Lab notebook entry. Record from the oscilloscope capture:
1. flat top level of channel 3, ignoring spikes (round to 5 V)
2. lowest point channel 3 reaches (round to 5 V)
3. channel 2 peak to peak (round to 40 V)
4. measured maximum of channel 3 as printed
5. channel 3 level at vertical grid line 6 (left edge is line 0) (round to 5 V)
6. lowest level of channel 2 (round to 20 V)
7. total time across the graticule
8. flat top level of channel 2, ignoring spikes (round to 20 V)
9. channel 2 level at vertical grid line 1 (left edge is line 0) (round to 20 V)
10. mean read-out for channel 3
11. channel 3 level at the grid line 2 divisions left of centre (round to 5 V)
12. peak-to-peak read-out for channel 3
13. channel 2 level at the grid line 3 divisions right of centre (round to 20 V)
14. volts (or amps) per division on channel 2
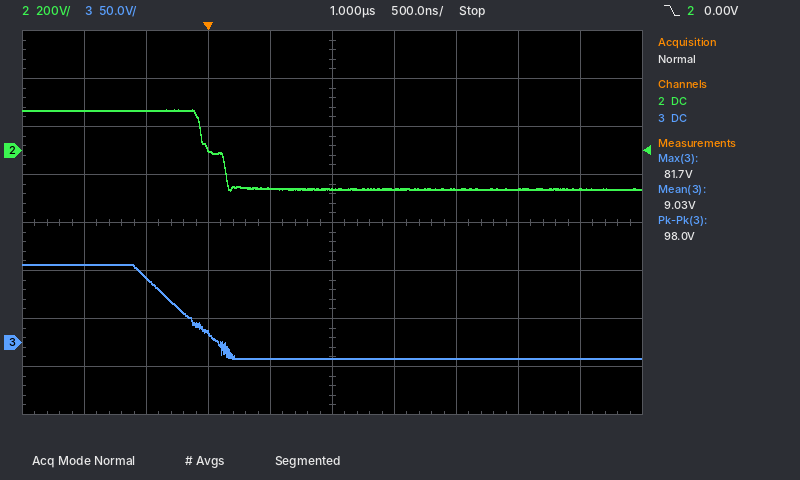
80 V
-15 V
320 V
81.7 V
-15 V
-160 V
5 µs
160 V
160 V
9.03 V
10 V
98.0 V
-160 V
200 V
